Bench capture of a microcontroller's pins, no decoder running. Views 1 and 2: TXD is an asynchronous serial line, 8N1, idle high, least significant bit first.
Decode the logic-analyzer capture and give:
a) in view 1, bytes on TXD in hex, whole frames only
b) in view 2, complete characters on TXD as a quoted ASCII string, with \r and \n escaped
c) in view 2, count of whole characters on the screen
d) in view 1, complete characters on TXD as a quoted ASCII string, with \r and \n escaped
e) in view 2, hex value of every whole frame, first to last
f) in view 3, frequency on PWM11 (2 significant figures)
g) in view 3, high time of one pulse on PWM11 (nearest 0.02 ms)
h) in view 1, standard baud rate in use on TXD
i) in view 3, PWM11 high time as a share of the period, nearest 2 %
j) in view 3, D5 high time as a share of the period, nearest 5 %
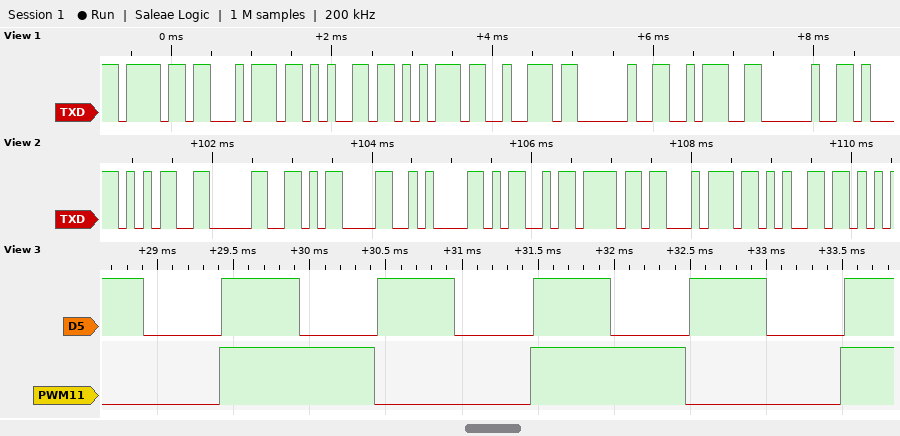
6F 74 65 75 72 20 3A 20
"50\r\nMote"
8
"oteur : "
35 30 0D 0A 4D 6F 74 65
490 Hz
1.02 ms
9600 baud
50 %
50 %
